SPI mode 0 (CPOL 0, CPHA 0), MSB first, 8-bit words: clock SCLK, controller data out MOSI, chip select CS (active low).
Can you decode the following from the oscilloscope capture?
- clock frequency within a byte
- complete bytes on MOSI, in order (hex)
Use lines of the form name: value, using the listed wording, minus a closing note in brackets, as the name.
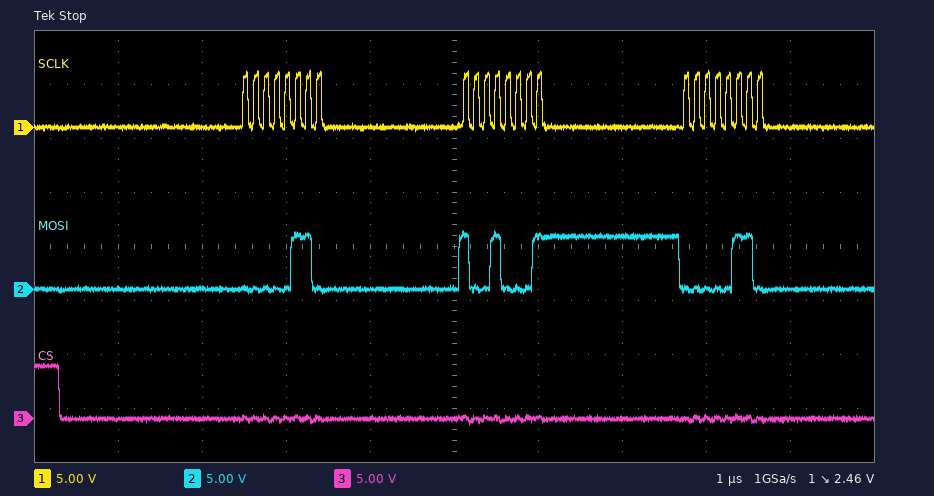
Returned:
clock frequency within a byte: 8 MHz
complete bytes on MOSI, in order: 06 91 06
